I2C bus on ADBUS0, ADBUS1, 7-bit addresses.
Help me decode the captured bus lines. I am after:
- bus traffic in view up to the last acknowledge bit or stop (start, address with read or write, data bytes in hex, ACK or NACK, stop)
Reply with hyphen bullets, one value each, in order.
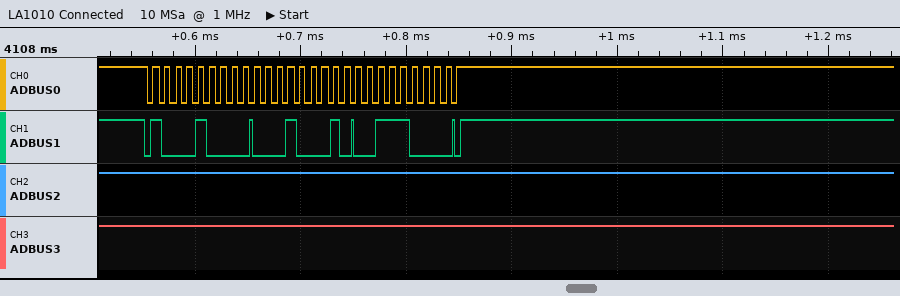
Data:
- start, address 44 write ACK, 11 ACK, 38 ACK, stop
